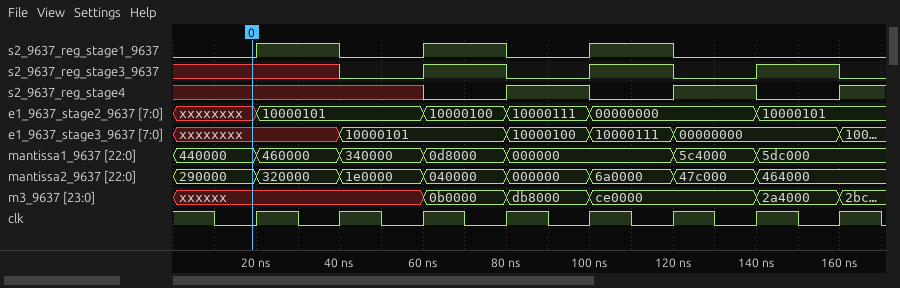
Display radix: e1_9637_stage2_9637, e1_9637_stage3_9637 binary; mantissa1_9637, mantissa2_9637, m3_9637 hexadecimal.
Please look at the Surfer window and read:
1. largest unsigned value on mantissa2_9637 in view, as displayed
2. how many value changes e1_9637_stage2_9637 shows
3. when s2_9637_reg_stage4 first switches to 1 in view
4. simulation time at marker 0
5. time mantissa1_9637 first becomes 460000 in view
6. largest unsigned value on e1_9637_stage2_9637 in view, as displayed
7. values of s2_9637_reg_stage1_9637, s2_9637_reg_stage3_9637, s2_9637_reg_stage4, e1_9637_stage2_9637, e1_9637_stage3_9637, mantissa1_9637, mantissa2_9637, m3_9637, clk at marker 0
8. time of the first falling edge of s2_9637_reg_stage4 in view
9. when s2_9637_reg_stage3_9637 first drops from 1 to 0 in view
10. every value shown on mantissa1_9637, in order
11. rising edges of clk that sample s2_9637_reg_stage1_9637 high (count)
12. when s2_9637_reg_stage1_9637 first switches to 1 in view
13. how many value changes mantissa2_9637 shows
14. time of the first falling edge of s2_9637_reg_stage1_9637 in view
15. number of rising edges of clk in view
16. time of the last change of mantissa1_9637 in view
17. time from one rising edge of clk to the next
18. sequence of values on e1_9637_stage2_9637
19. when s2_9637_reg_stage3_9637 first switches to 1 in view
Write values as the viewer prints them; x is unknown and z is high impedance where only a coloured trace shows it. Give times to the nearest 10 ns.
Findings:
6a0000
5
80 ns
20 ns
20 ns
10000111
s2_9637_reg_stage1_9637=0, s2_9637_reg_stage3_9637=x, s2_9637_reg_stage4=x, e1_9637_stage2_9637=xxxxxxxx, e1_9637_stage3_9637=xxxxxxxx, mantissa1_9637=440000, mantissa2_9637=290000, m3_9637=xxxxxx, clk=0
100 ns
80 ns
440000, 460000, 340000, 0d8000, 000000, 5c4000, 5dc000
3
20 ns
7
40 ns
8
140 ns
20 ns
xxxxxxxx, 10000101, 10000100, 10000111, 00000000, 10000101
60 ns
